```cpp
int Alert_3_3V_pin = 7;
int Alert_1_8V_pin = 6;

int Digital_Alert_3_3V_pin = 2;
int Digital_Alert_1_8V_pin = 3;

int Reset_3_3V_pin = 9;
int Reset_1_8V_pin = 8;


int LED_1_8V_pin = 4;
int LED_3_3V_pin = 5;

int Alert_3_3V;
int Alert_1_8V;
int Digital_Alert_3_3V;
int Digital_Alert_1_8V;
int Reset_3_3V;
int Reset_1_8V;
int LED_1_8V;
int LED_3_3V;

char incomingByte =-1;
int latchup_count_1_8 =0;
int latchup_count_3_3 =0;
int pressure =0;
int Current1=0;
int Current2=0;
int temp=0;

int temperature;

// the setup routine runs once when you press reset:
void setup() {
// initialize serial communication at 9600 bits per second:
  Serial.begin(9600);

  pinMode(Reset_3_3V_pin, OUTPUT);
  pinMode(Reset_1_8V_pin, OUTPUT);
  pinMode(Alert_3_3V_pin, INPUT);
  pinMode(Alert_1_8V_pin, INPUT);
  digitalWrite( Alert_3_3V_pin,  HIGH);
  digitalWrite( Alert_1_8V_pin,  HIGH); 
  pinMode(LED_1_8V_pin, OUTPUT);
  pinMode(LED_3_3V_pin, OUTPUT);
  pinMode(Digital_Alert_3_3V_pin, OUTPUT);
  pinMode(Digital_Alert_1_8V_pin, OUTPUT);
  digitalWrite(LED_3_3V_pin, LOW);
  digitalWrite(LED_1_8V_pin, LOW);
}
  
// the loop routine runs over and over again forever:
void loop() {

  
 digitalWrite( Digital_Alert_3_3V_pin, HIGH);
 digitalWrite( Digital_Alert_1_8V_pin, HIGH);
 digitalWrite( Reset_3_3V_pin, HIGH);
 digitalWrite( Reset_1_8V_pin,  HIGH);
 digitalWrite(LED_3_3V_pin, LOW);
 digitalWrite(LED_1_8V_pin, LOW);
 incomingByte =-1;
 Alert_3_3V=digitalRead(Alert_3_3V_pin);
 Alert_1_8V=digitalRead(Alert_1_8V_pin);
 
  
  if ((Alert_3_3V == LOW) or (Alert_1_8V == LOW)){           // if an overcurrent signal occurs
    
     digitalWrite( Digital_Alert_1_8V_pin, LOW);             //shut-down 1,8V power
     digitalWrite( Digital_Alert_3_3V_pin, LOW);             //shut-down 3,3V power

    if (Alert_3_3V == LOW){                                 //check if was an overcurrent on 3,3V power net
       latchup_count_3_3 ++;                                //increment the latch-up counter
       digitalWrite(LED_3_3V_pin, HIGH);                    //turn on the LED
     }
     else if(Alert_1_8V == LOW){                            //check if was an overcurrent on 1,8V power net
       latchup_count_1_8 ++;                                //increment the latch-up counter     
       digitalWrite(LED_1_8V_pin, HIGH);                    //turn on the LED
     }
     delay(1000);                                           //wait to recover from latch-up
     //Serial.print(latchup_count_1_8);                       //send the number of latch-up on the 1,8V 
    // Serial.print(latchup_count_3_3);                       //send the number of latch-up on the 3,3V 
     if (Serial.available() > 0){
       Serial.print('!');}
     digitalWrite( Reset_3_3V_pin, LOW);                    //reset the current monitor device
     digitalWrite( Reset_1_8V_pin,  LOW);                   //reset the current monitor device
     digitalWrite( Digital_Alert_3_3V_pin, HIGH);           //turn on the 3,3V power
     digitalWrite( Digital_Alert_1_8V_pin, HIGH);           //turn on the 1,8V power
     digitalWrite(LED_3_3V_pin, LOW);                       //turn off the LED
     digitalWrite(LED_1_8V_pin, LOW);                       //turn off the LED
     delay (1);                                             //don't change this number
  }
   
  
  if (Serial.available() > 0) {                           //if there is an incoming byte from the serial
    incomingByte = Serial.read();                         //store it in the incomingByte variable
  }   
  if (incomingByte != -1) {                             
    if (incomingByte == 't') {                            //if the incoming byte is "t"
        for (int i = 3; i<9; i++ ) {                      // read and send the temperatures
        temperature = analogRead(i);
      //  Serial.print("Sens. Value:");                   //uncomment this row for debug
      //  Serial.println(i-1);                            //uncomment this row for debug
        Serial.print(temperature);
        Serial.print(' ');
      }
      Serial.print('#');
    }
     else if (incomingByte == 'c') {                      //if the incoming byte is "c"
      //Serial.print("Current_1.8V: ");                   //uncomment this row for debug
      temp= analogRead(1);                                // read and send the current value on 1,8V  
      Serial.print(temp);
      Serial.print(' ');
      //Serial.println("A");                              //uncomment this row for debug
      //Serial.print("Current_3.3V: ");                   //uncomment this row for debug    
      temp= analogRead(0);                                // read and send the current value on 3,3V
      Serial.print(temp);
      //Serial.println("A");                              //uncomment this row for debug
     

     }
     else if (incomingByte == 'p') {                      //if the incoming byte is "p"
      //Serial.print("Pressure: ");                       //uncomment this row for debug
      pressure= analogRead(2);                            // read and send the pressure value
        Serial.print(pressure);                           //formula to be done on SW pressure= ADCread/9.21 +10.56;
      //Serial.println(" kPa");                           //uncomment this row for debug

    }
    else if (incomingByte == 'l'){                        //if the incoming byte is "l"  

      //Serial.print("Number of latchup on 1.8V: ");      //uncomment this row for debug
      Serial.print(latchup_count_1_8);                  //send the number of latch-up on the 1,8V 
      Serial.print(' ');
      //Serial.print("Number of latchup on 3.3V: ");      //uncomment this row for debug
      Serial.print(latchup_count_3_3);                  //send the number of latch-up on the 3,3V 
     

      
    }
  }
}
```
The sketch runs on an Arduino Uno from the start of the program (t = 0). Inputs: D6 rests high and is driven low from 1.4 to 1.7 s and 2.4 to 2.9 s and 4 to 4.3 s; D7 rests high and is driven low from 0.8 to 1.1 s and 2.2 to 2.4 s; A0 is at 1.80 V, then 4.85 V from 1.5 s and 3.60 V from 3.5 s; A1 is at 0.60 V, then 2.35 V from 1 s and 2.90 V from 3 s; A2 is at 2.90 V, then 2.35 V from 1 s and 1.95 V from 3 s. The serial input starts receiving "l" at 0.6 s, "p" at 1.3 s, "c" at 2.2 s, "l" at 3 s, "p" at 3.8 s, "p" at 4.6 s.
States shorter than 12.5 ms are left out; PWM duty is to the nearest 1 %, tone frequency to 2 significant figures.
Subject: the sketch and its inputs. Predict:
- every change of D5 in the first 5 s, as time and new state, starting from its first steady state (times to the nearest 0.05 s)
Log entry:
0 s low; 0.8 s high; 1.8 s low; 2.2 s high; 3.2 s low
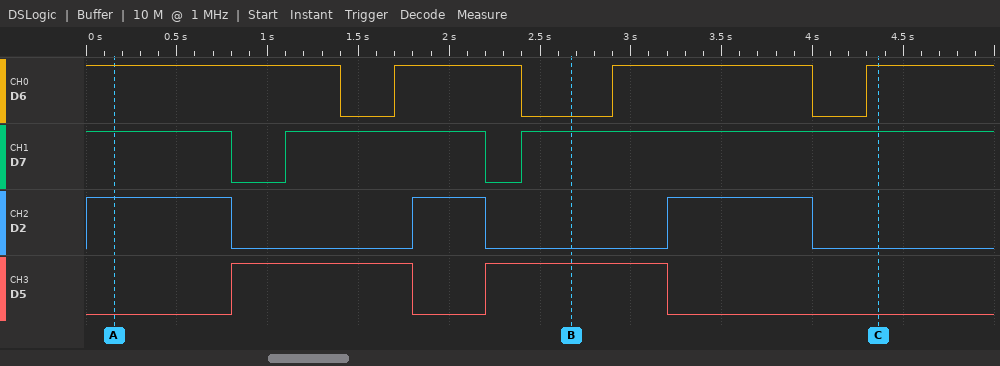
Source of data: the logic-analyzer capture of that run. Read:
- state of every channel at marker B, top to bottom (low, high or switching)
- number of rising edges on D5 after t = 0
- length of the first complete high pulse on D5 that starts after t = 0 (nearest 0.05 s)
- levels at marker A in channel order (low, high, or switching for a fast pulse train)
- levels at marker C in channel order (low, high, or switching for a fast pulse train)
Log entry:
D6 low, D7 high, D2 low, D5 high
2
1.00 s
D6 high, D7 high, D2 high, D5 low
D6 high, D7 high, D2 low, D5 low
